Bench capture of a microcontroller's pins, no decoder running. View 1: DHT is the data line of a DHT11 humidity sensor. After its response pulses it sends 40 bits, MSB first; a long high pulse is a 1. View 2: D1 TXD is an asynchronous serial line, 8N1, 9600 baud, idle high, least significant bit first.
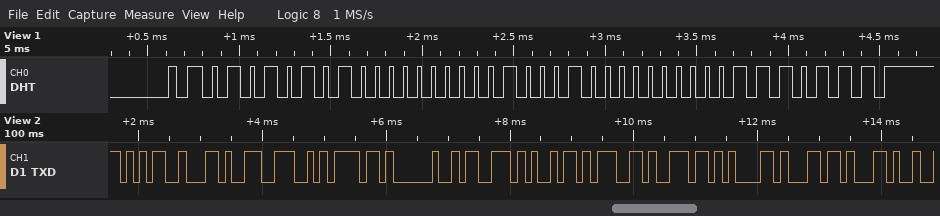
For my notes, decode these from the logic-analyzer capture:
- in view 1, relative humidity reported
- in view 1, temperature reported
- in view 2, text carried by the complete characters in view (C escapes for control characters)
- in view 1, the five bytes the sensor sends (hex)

85 %
34.0 °C
"5,No signal,"
55 00 22 00 77
